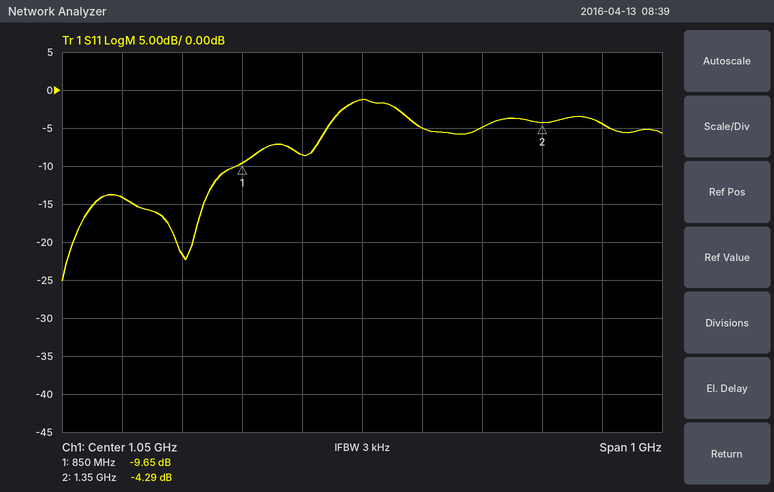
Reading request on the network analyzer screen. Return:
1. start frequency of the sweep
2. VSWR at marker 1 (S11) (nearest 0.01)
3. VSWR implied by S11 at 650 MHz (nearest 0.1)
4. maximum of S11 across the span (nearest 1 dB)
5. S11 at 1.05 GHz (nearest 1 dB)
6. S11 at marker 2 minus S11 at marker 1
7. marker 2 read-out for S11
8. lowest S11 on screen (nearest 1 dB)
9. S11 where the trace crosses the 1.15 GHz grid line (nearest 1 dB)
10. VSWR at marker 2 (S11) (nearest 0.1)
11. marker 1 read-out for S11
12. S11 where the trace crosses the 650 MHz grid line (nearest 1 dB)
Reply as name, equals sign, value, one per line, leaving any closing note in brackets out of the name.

start frequency of the sweep = 550 MHz
VSWR at marker 1 (S11) = 1.98
VSWR implied by S11 at 650 MHz = 1.5
maximum of S11 across the span = -1 dB
S11 at 1.05 GHz = -1 dB
S11 at marker 2 minus S11 at marker 1 = 5.36 dB
marker 2 read-out for S11 = -4.29 dB
lowest S11 on screen = -25 dB
S11 where the trace crosses the 1.15 GHz grid line = -5 dB
VSWR at marker 2 (S11) = 4.1
marker 1 read-out for S11 = -9.65 dB
S11 where the trace crosses the 650 MHz grid line = -14 dB
